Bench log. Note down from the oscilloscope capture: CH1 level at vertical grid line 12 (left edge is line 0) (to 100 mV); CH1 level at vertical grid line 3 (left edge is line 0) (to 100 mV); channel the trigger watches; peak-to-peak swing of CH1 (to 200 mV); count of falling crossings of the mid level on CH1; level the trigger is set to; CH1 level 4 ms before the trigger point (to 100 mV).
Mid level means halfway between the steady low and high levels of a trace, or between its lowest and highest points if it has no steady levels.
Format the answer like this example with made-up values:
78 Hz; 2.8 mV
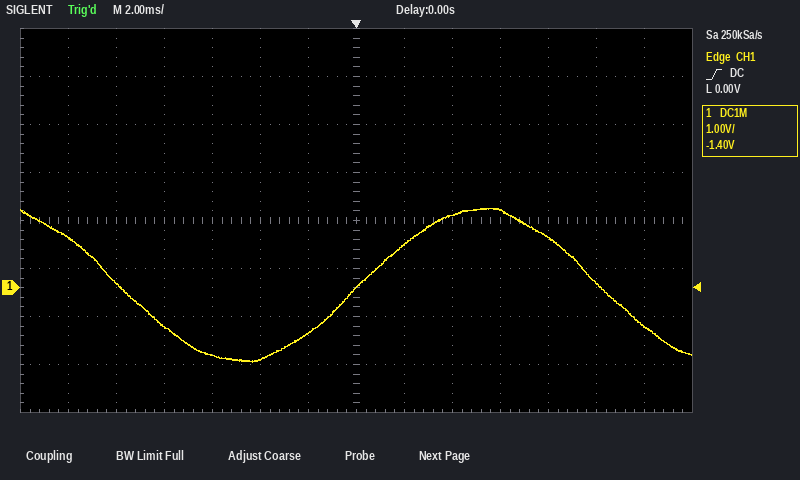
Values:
100 mV; -800 mV; CH1; 3.2 V; 2; 0.00 V; -1.5 V
